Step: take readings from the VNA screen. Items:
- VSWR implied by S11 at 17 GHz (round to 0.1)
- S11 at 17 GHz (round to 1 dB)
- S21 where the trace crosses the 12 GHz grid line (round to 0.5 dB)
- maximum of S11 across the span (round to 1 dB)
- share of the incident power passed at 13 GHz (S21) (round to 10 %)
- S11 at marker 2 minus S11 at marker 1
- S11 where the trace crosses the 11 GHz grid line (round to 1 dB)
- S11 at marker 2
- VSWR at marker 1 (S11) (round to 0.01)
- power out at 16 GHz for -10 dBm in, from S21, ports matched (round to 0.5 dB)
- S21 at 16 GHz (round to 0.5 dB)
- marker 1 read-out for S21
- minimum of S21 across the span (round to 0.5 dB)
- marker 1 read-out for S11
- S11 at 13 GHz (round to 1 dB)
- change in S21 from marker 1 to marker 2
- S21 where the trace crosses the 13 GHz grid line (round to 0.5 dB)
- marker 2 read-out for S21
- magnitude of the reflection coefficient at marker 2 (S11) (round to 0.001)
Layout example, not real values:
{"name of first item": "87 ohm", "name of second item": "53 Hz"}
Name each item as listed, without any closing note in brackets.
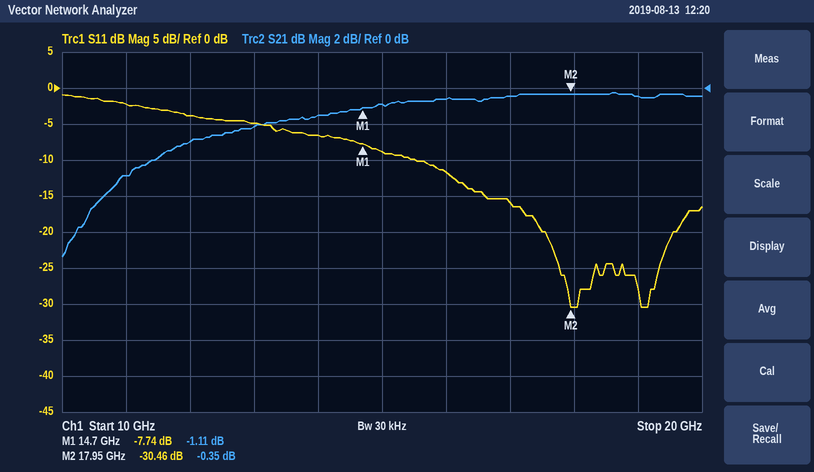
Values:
{"VSWR implied by S11 at 17 GHz": "1.4", "S11 at 17 GHz": "-16 dB", "S21 where the trace crosses the 12 GHz grid line": "-3.0 dB", "maximum of S11 across the span": "-1 dB", "share of the incident power passed at 13 GHz (S21)": "60 %", "S11 at marker 2 minus S11 at marker 1": "-22.72 dB", "S11 where the trace crosses the 11 GHz grid line": "-2 dB", "S11 at marker 2": "-30.46 dB", "VSWR at marker 1 (S11)": "2.39", "power out at 16 GHz for -10 dBm in, from S21, ports matched": "-10.5 dBm", "S21 at 16 GHz": "-0.5 dB", "marker 1 read-out for S21": "-1.11 dB", "minimum of S21 across the span": "-9.5 dB", "marker 1 read-out for S11": "-7.74 dB", "S11 at 13 GHz": "-5 dB", "change in S21 from marker 1 to marker 2": "0.76 dB", "S21 where the trace crosses the 13 GHz grid line": "-2.0 dB", "marker 2 read-out for S21": "-0.35 dB", "magnitude of the reflection coefficient at marker 2 (S11)": "0.030"}
